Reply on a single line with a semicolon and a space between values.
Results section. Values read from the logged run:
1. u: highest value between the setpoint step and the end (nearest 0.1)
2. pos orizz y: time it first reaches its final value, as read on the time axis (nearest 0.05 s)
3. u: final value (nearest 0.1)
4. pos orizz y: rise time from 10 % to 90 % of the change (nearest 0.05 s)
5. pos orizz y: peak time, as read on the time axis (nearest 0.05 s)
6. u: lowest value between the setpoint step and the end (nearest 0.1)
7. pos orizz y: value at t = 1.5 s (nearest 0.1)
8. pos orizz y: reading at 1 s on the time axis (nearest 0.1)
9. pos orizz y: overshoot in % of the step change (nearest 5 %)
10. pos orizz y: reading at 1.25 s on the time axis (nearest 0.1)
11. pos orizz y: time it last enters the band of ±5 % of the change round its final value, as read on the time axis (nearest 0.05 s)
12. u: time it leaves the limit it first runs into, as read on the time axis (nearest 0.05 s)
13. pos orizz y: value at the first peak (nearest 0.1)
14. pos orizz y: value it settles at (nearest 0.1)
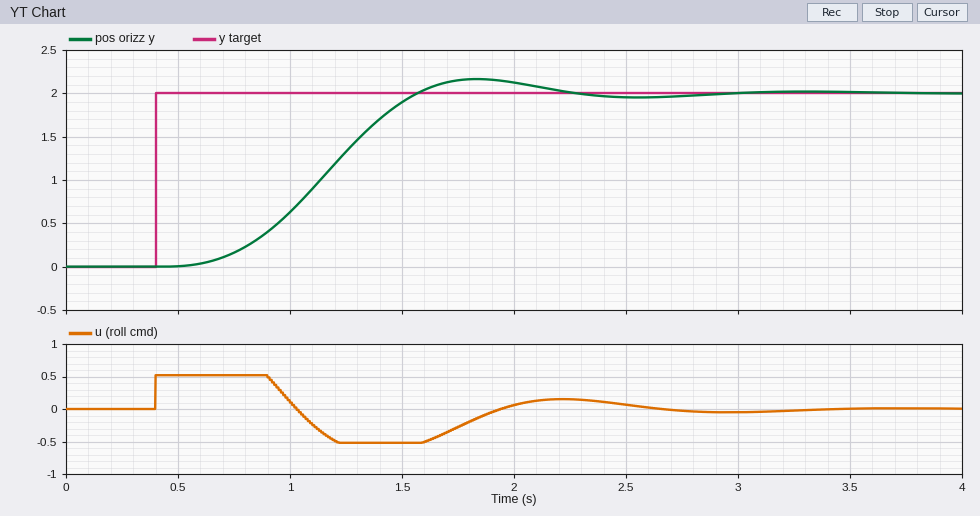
0.5; 1.55 s; 0.0; 0.65 s; 1.85 s; -0.5; 1.9; 0.6; 10 %; 1.3; 2.05 s; 0.90 s; 2.2; 2.0
